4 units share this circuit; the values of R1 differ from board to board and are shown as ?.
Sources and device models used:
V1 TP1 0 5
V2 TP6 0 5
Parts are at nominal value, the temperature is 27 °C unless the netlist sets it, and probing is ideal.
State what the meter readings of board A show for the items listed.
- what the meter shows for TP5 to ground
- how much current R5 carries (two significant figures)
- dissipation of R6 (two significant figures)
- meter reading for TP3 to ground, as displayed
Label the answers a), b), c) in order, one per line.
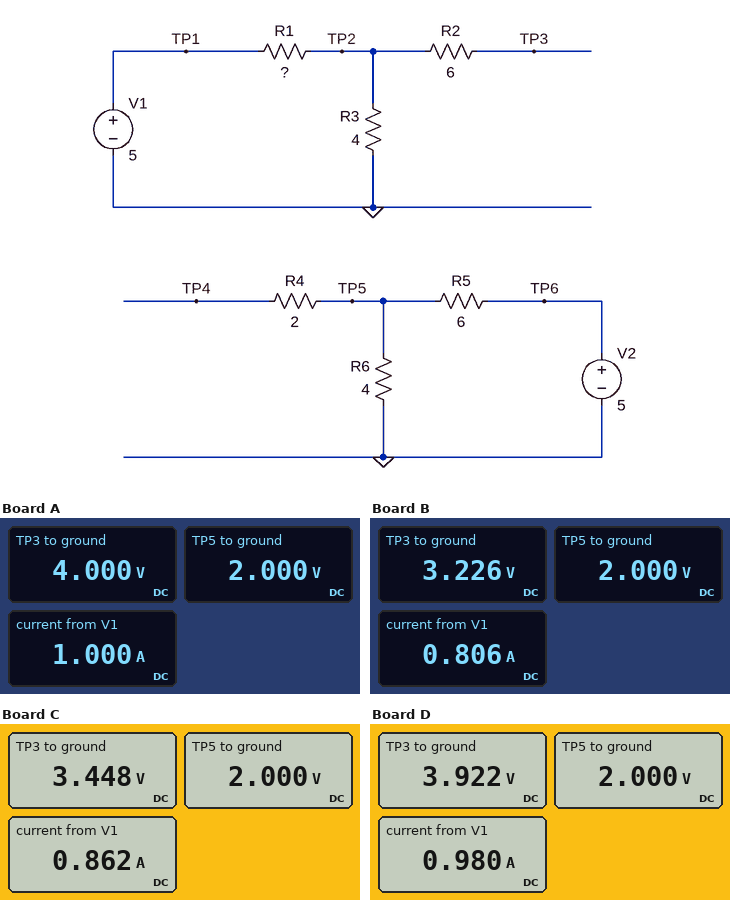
a) 2.000 V
b) 500 mA
c) 1.0 W
d) 4.000 V
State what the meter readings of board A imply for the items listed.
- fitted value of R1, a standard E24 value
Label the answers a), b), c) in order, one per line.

a) 1 Ω
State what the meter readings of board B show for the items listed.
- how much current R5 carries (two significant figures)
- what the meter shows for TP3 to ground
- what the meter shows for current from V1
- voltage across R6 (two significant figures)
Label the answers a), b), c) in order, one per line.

a) 500 mA
b) 3.226 V
c) 0.806 A
d) 2.0 V
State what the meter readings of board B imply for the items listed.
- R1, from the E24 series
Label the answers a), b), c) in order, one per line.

a) 2.2 Ω
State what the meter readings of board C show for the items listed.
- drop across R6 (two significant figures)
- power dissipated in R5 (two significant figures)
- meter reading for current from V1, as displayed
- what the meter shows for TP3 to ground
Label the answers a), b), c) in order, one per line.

a) 2.0 V
b) 1.5 W
c) 0.862 A
d) 3.448 V
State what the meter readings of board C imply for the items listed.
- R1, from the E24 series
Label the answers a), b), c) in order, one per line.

a) 1.8 Ω
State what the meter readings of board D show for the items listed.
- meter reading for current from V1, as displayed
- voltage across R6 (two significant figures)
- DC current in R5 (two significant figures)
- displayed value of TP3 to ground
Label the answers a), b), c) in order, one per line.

a) 0.980 A
b) 2.0 V
c) 500 mA
d) 3.922 V
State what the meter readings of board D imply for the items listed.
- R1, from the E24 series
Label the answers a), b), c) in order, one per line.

a) 1.1 Ω
